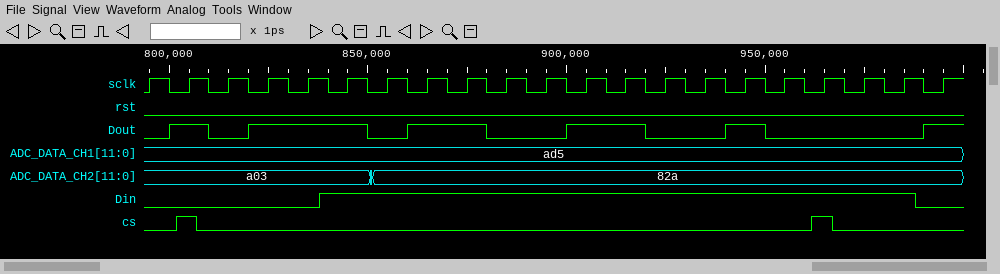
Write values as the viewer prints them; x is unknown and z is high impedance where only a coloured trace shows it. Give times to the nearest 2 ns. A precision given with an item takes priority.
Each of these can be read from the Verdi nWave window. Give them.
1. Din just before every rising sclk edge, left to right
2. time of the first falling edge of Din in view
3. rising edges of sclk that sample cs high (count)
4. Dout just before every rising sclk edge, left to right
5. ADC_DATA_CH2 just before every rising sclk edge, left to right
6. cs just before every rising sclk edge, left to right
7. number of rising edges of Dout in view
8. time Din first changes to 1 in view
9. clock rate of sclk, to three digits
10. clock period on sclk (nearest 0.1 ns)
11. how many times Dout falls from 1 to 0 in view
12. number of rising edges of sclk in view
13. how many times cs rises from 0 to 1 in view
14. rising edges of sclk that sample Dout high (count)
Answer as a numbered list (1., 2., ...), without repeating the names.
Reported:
1. 0 0 0 0 0 1 1 1 1 1 1 1 1 1 1 1 1 1 1 1 0
2. 988 ns
3. 2
4. 0 1 0 1 1 1 0 1 1 0 0 1 1 0 0 1 0 0 0 0 1
5. a03, a03, a03, a03, a03, a03, 82a, 82a, 82a, 82a, 82a, 82a, 82a, 82a, 82a, 82a, 82a, 82a, 82a, 82a, 82a
6. 0 1 0 0 0 0 0 0 0 0 0 0 0 0 0 0 0 1 0 0 0
7. 6
8. 838 ns
9. 100 MHz
10. 10 ns
11. 5
12. 21
13. 2
14. 10
